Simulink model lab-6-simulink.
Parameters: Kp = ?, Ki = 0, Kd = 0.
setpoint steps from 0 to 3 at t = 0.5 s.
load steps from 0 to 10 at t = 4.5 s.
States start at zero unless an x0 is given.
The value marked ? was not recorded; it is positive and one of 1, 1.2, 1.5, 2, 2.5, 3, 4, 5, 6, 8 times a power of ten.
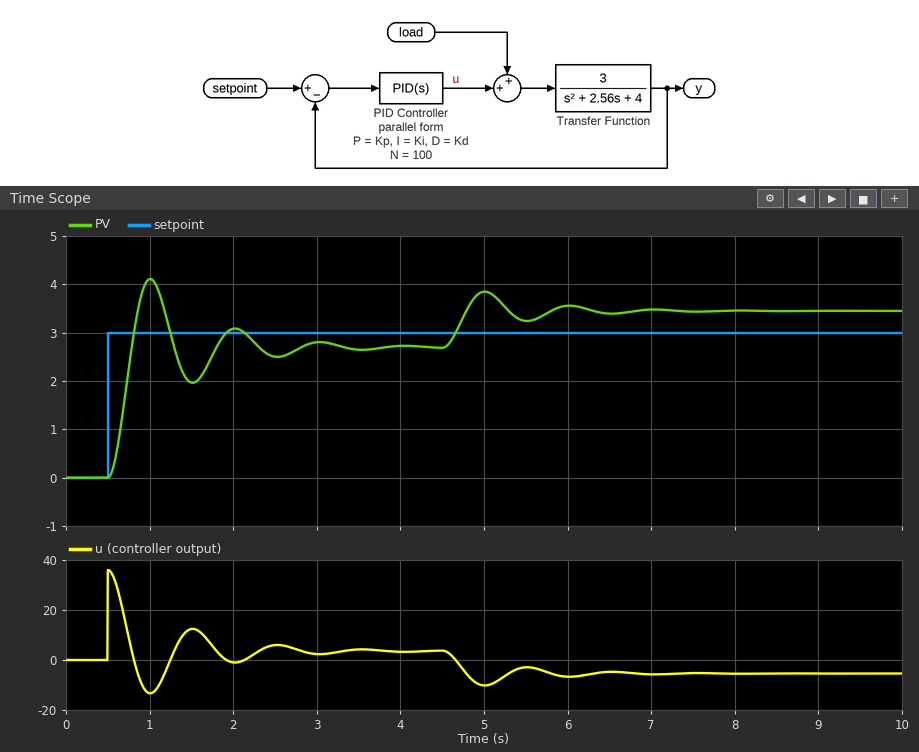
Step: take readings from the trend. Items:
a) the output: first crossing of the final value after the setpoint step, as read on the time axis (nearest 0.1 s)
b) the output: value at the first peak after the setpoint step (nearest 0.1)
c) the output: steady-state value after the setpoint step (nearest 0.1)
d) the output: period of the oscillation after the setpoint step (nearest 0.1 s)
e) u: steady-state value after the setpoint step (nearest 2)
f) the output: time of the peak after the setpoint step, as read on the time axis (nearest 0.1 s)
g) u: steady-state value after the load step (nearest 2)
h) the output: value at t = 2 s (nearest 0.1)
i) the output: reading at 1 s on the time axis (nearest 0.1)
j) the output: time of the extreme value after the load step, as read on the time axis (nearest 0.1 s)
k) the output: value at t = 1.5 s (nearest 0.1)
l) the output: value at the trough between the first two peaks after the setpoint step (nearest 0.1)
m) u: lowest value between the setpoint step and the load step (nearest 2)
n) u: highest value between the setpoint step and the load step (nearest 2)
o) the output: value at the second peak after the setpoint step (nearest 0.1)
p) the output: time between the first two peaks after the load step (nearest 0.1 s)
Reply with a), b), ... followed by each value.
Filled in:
a) 0.8 s
b) 4.1
c) 2.7
d) 1.0 s
e) 4
f) 1.0 s
g) -6
h) 3.1
i) 4.1
j) 5.0 s
k) 2.0
l) 2.0
m) -14
n) 36
o) 3.1
p) 1.0 s
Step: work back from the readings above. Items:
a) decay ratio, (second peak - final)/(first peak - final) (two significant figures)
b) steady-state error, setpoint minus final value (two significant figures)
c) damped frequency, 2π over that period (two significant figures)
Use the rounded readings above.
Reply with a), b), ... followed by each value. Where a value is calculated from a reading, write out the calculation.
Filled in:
a) (3.1 - 2.7) / (4.1 - 2.7) = 0.29
b) 3 - 2.7 = 0.30
c) 2π / 1 = 6.3 rad/s
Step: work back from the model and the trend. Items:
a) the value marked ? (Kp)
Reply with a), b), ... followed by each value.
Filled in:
a) 12
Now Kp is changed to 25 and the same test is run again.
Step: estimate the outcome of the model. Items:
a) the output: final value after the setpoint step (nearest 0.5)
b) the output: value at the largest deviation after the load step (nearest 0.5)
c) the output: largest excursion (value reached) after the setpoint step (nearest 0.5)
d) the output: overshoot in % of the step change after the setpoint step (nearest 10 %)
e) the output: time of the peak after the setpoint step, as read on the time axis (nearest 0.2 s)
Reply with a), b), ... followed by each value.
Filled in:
a) 3.0
b) 3.5
c) 4.5
d) 60 %
e) 0.8 s
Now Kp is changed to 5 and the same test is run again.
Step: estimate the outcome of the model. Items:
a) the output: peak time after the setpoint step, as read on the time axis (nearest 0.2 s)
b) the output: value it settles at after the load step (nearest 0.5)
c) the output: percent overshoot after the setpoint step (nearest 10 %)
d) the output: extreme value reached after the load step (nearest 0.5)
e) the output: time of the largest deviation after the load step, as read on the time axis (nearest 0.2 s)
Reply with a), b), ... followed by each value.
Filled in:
a) 1.2 s
b) 4.0
c) 40 %
d) 4.5
e) 5.2 s
